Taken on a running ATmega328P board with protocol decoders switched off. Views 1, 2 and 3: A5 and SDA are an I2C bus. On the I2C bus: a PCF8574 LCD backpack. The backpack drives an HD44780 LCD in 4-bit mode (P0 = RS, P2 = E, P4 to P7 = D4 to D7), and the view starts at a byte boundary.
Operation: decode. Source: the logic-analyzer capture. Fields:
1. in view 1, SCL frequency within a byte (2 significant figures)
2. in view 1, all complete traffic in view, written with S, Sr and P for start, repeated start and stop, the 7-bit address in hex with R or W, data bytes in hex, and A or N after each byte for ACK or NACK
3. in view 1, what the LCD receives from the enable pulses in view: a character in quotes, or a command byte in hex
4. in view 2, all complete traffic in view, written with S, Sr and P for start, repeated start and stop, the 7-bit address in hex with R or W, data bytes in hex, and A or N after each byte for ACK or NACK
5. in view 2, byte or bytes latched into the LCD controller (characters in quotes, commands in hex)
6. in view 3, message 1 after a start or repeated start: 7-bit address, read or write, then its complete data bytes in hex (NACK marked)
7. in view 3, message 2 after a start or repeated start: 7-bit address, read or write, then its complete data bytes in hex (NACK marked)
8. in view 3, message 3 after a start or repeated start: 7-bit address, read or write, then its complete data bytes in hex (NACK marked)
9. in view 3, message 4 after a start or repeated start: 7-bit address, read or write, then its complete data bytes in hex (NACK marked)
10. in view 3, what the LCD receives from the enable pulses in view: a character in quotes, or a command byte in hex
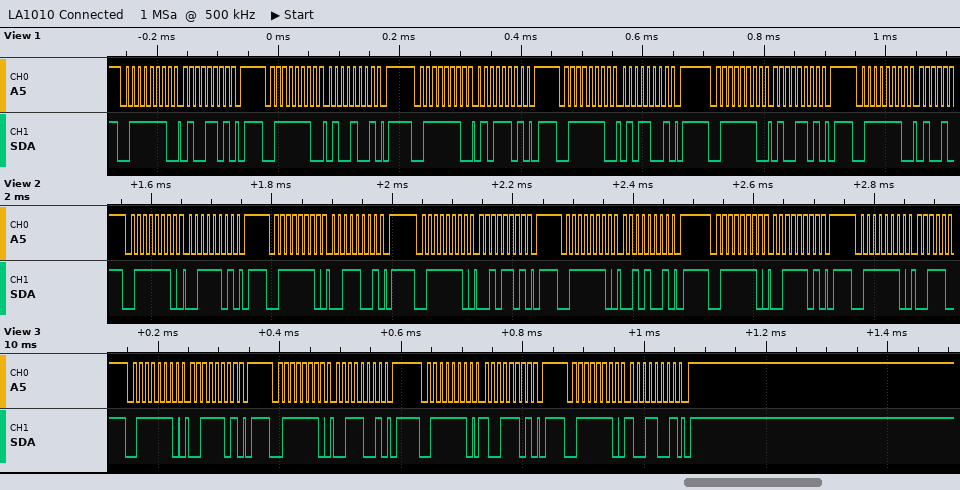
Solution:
100 kHz
S 3FW A 4D A P S 3FW A 49 A P S 3FW A 5D A P S 3FW A 59 A P S 3FW A 4D A P S 3FW A
'E'
S 3FW A 3D A P S 3FW A 39 A P S 3FW A 2D A P S 3FW A 29 A P S 3FW A 3D A P S 3FW A
'2'
0x3F write: 3D
0x3F write: 39
0x3F write: 9D
0x3F write: 99
'9'
